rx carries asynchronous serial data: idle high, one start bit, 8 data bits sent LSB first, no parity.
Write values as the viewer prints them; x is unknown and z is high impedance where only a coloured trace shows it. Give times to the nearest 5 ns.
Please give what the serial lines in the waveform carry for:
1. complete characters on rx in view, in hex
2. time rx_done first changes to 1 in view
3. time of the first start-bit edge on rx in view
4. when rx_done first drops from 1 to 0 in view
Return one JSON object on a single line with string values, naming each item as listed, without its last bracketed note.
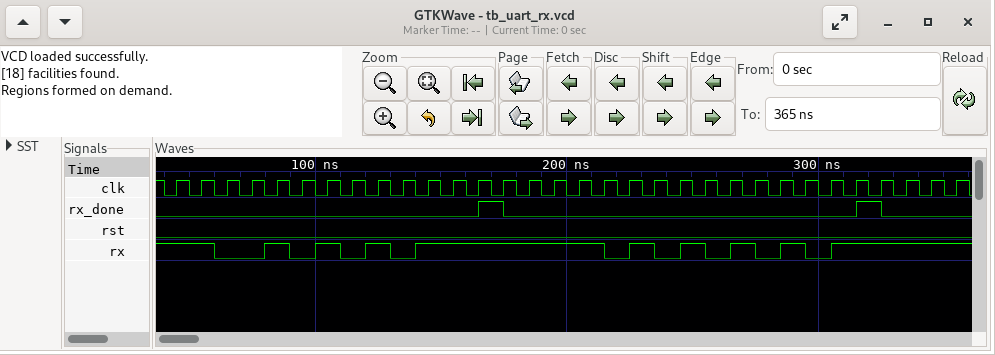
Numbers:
{"complete characters on rx in view, in hex": "AA, 55", "time rx_done first changes to 1 in view": "165 ns", "time of the first start-bit edge on rx in view": "60 ns", "when rx_done first drops from 1 to 0 in view": "175 ns"}
